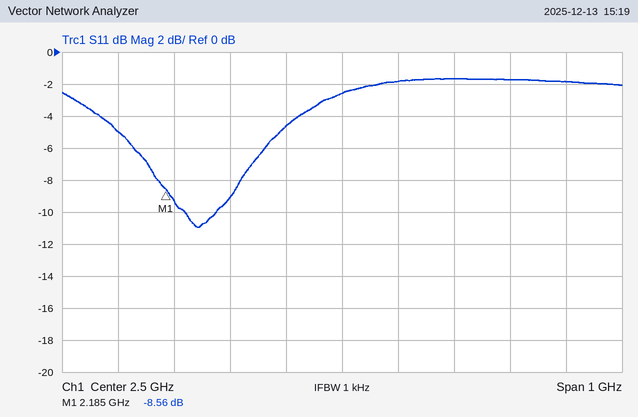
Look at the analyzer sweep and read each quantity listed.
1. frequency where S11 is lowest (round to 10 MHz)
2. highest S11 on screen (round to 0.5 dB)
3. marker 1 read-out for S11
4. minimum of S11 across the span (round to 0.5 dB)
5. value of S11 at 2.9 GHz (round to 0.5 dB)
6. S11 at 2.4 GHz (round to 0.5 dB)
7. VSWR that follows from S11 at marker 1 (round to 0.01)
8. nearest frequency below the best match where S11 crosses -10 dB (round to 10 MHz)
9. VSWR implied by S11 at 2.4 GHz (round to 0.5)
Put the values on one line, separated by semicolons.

2.24 GHz; -1.5 dB; -8.56 dB; -11.0 dB; -2.0 dB; -4.5 dB; 2.19; 2.22 GHz; 4.0
